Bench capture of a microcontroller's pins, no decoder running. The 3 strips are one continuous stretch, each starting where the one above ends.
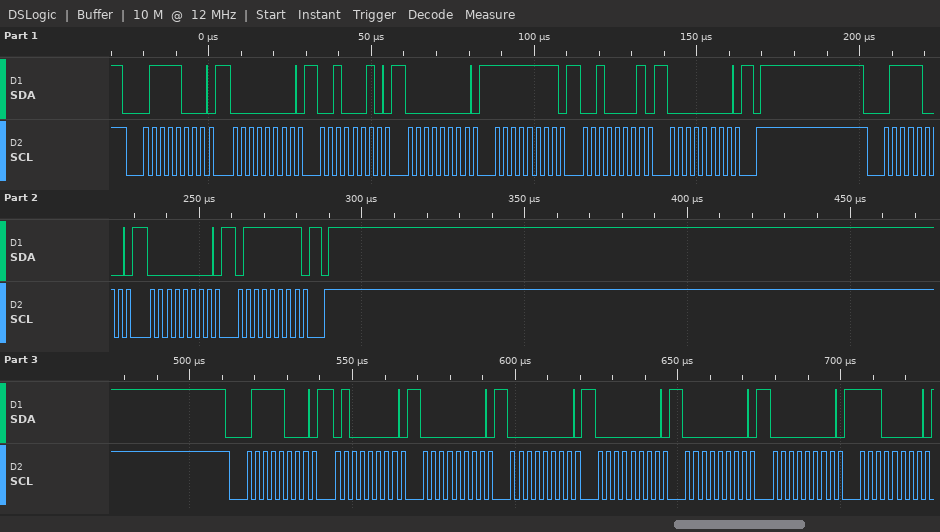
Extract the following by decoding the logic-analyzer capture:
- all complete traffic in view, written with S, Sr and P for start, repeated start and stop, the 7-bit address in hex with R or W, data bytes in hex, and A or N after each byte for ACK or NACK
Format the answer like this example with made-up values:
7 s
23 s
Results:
S 3CW A 00 A 22 A 00 A FF A 21 A 00 A P S 3CW A 00 A 7F A P S 3CW A 40 A 00 A 00 A 00 A 00 A 00 A E0 A
